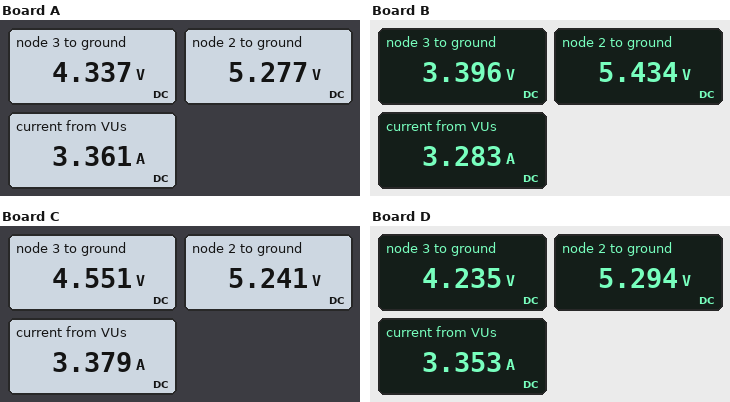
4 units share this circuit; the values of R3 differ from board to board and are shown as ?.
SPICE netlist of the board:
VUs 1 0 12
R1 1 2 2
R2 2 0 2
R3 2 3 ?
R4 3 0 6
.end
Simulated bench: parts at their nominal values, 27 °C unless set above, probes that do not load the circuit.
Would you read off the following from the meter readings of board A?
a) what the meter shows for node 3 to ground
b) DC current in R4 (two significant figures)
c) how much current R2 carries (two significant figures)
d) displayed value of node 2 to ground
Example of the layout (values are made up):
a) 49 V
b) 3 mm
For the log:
a) 4.337 V
b) 720 mA
c) 2.6 A
d) 5.277 V
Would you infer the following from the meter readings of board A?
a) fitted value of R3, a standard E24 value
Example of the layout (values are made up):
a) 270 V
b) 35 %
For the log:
a) 1.3 Ω
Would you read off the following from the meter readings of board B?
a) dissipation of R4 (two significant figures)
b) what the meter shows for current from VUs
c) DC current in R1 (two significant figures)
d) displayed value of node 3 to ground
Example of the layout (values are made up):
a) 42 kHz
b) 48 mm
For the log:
a) 1.9 W
b) 3.283 A
c) 3.3 A
d) 3.396 V
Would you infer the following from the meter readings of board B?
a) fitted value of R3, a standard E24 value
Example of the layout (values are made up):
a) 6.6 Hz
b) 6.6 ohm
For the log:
a) 3.6 Ω
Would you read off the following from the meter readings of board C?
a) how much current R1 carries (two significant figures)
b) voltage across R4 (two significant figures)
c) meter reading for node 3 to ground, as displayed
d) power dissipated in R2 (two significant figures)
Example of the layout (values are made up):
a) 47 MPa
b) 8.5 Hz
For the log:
a) 3.4 A
b) 4.6 V
c) 4.551 V
d) 14 W
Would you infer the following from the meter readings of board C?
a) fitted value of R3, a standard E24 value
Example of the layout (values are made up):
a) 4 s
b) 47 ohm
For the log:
a) 0.91 Ω
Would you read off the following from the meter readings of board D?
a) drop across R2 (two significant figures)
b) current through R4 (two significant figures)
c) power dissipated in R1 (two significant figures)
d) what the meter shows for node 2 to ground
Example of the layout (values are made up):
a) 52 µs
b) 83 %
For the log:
a) 5.3 V
b) 710 mA
c) 22 W
d) 5.294 V
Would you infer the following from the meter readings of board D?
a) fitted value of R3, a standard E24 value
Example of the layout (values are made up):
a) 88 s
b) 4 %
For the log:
a) 1.5 Ω
